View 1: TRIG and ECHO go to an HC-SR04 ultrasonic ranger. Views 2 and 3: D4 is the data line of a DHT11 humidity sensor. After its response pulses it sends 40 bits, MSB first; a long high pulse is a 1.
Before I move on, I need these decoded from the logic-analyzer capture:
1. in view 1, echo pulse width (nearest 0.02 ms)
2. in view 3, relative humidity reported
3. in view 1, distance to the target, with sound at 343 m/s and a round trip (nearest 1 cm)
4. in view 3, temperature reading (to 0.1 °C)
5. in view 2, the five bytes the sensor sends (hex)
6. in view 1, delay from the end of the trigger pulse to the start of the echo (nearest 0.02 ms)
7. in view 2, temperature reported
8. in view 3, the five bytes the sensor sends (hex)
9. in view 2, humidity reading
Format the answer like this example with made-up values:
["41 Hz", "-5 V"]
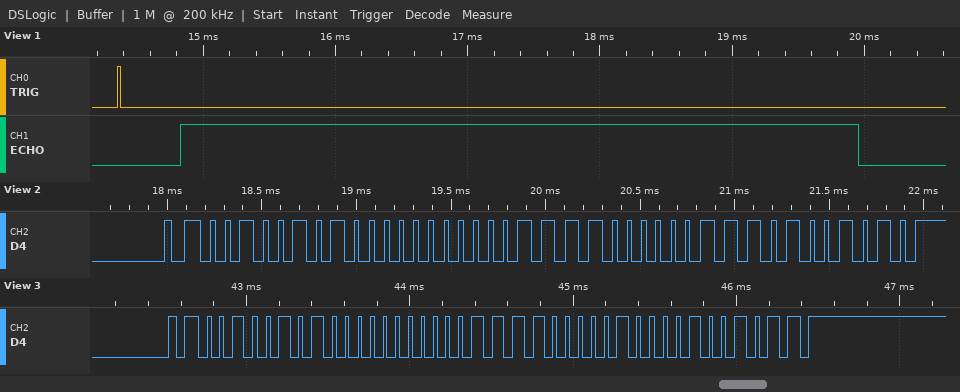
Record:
["5.12 ms", "37 %", "88 cm", "30.8 °C", "25 00 1E 07 4A", "0.46 ms", "30.7 °C", "25 00 1E 08 4B", "37 %"]
